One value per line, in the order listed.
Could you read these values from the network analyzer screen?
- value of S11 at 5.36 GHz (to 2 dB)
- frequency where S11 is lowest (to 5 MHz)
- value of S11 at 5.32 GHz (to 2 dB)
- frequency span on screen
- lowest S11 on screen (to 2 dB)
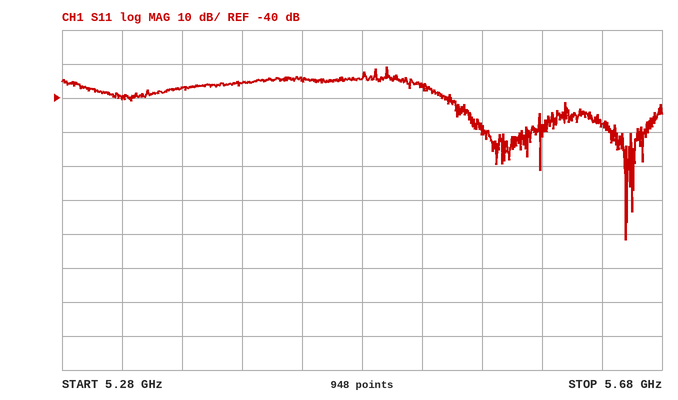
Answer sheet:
-36 dB
5.655 GHz
-40 dB
400 MHz
-82 dB
